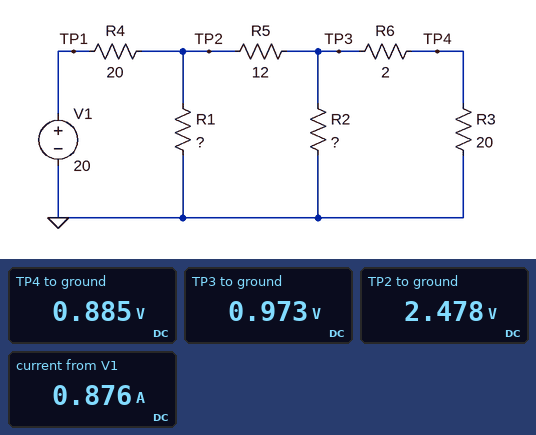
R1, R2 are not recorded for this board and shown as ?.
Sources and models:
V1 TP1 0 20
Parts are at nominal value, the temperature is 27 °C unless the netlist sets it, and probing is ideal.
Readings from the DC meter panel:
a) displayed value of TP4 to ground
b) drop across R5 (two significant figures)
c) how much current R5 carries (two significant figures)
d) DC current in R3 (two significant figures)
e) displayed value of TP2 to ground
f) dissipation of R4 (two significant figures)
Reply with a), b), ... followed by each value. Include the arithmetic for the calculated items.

a) 0.885 V
b) 2.478 V - 973 mV = 1.5 V
c) (2.478 V - 973 mV) / 12 Ω = 130 mA
d) (885 mV) / 20 Ω = 44 mA
e) 2.478 V
f) (20 V - 2.478 V)^2 / 20 Ω = 15 W
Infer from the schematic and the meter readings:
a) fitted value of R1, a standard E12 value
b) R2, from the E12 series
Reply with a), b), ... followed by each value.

a) 3.3 Ω
b) 12 Ω
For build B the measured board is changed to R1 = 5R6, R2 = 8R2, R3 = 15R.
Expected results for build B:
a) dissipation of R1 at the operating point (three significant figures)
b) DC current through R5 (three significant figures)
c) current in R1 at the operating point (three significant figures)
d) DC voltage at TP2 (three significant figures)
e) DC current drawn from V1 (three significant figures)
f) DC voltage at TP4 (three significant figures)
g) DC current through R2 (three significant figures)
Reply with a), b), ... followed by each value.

a) 2.19 W
b) 200 mA
c) 625 mA
d) 3.50 V
e) 825 mA
f) 975 mV
g) 135 mA
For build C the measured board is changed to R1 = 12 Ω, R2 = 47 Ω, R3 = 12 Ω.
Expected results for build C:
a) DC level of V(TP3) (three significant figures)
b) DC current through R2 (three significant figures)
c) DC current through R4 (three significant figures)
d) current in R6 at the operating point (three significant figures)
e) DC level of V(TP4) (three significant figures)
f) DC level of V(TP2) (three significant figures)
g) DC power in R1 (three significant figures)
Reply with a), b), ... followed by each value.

a) 2.67 V
b) 56.8 mA
c) 718 mA
d) 191 mA
e) 2.29 V
f) 5.64 V
g) 2.65 W
